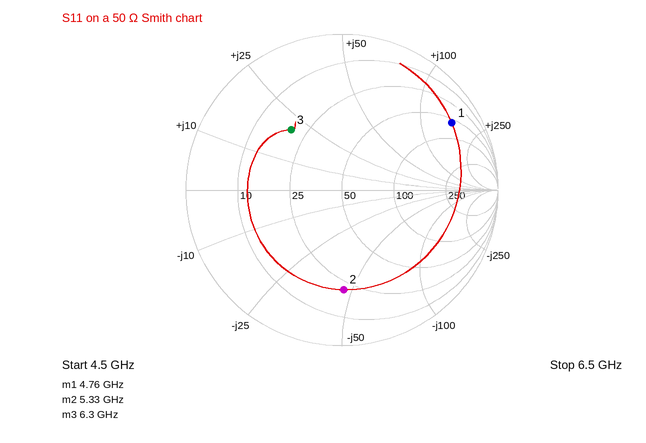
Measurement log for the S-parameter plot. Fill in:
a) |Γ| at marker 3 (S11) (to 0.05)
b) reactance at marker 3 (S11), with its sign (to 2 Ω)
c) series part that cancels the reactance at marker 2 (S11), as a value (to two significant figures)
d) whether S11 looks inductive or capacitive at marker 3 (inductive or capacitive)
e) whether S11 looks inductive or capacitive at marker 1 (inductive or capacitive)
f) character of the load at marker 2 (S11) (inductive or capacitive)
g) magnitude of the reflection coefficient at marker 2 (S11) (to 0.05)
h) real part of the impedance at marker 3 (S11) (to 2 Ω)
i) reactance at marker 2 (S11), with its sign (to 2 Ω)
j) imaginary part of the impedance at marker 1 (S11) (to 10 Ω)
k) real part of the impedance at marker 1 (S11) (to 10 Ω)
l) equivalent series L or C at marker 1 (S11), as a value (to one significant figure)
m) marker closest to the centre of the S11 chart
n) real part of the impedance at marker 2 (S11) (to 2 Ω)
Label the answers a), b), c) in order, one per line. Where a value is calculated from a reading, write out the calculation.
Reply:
a) 0.50
b) +20 Ω
c) L = 46 Ω/(2π × 5.33 GHz) ≈ 1.4 nH
d) inductive
e) inductive
f) capacitive
g) 0.65
h) 20 Ω
i) -46 Ω
j) +160 Ω
k) 60 Ω
l) L = 160 Ω/(2π × 4.76 GHz) ≈ 5 nH
m) marker 3
n) 22 Ω
